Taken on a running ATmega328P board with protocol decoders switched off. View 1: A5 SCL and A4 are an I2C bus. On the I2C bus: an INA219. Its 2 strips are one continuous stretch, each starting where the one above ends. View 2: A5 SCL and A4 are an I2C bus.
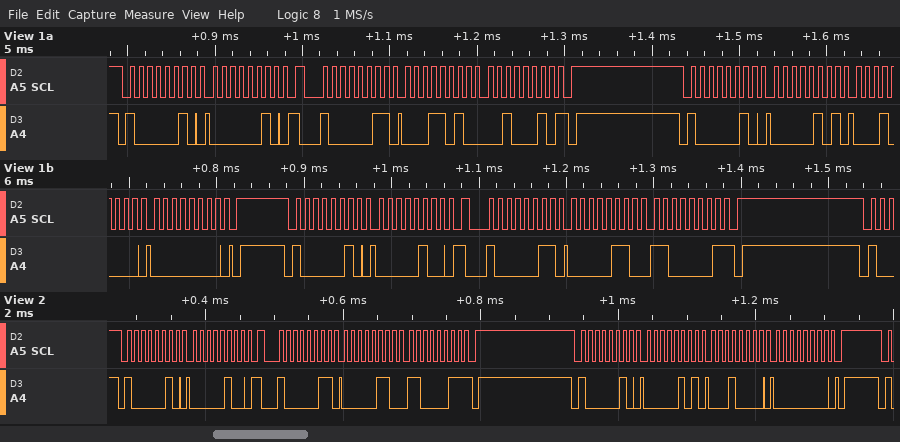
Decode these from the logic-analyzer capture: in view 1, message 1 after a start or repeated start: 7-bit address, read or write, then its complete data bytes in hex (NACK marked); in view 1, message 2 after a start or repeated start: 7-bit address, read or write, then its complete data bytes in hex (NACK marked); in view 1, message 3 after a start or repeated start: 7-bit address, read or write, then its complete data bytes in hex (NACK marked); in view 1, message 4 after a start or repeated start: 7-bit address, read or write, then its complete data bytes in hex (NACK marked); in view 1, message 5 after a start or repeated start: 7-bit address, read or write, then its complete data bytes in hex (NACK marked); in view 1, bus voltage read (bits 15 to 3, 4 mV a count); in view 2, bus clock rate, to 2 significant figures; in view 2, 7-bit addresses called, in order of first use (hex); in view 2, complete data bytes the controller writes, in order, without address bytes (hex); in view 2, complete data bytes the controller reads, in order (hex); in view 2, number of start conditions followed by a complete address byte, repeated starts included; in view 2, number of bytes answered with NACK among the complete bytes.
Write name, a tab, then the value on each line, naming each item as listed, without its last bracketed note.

in view 1, message 1 after a start or repeated start: 7-bit address, read or write, then its complete data bytes in hex	0x41 write: 02
in view 1, message 2 after a start or repeated start: 7-bit address, read or write, then its complete data bytes in hex	0x41 read: 1A 22 NACK
in view 1, message 3 after a start or repeated start: 7-bit address, read or write, then its complete data bytes in hex	0x41 write: 05 10 00
in view 1, message 4 after a start or repeated start: 7-bit address, read or write, then its complete data bytes in hex	0x41 write: 04
in view 1, message 5 after a start or repeated start: 7-bit address, read or write, then its complete data bytes in hex	0x41 read: 06 C1 NACK
in view 1, bus voltage read	3.344 V
in view 2, bus clock rate, to 2 significant figures	100 kHz
in view 2, 7-bit addresses called, in order of first use	0x41
in view 2, complete data bytes the controller writes, in order, without address bytes	04 05 10 00
in view 2, complete data bytes the controller reads, in order	06 C3
in view 2, number of start conditions followed by a complete address byte, repeated starts included	3
in view 2, number of bytes answered with NACK among the complete bytes	1
